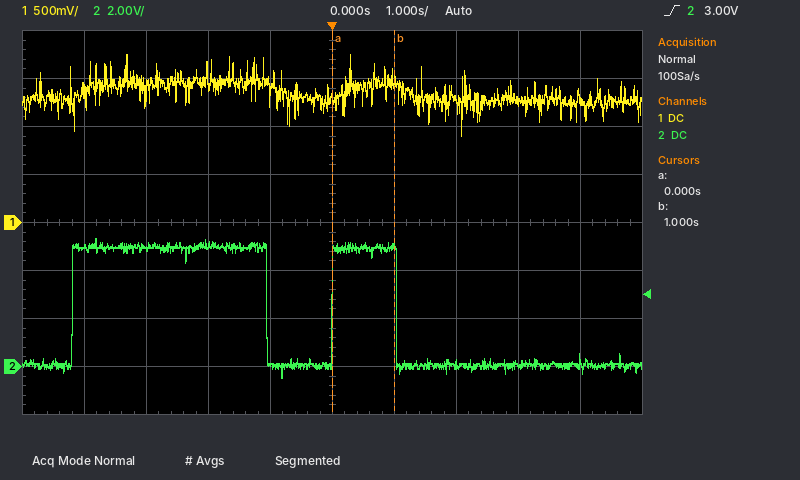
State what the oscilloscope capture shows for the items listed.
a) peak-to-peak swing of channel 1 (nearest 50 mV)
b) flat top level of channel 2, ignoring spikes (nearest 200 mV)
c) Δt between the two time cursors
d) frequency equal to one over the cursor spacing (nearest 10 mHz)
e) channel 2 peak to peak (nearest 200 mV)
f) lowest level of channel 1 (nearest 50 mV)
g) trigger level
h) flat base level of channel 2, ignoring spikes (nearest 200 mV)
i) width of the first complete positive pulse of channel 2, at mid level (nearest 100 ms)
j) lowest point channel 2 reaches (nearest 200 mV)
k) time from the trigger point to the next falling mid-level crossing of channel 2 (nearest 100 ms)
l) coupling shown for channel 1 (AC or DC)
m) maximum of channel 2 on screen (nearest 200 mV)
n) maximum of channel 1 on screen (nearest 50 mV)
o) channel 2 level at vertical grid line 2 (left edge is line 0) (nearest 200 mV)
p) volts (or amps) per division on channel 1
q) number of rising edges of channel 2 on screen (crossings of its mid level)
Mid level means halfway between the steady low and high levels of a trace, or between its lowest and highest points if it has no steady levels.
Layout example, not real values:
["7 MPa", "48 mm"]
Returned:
["850 mV", "5.0 V", "1.0 s", "1.00 Hz", "5.8 V", "900 mV", "3.00 V", "0.0 V", "3.1 s", "-400 mV", "1.0 s", "DC", "5.4 V", "1.75 V", "5.0 V", "500 mV", "2"]
